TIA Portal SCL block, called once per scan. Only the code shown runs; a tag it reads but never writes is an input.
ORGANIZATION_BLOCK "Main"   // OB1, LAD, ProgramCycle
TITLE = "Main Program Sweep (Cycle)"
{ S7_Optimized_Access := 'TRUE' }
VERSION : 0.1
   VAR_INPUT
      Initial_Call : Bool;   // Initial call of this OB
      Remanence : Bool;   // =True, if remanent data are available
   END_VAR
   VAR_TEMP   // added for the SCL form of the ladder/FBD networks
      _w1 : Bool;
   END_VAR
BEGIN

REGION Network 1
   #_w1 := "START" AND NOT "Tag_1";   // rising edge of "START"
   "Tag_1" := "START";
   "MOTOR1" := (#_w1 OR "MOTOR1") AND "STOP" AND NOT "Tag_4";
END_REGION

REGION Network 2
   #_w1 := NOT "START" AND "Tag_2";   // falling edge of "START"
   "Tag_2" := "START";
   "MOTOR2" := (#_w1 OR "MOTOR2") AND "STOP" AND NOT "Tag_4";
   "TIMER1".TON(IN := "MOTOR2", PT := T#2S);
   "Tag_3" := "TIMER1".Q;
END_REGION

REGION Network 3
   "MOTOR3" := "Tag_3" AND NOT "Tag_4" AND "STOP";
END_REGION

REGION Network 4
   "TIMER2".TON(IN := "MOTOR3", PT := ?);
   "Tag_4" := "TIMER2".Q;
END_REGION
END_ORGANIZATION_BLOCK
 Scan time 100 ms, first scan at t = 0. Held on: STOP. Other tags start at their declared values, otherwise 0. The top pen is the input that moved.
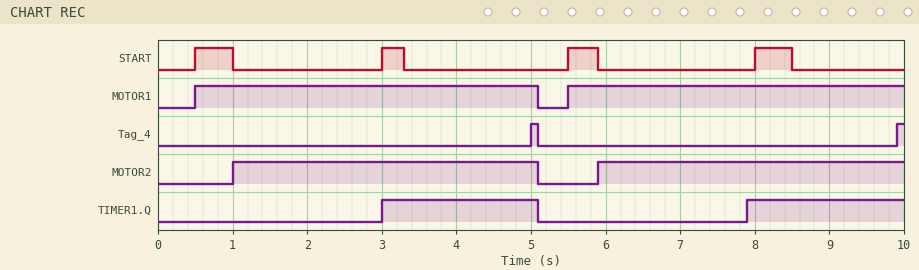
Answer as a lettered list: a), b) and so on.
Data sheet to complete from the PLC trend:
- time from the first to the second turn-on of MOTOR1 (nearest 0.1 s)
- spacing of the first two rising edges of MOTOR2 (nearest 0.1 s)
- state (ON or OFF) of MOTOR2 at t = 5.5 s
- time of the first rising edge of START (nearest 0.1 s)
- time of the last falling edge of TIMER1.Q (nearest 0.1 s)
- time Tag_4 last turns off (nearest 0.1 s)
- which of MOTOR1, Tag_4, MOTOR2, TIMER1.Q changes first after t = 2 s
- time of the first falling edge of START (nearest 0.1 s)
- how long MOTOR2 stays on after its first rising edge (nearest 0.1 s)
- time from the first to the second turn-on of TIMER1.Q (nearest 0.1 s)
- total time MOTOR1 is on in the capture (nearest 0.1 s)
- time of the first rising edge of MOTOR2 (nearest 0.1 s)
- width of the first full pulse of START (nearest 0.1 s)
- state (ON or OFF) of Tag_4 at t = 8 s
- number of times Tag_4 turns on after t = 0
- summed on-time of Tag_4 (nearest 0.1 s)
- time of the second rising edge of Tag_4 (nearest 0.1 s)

a) 5.0 s
b) 4.9 s
c) OFF
d) 0.5 s
e) 5.1 s
f) 5.1 s
g) TIMER1.Q
h) 1.0 s
i) 4.1 s
j) 4.9 s
k) 9.1 s
l) 1.0 s
m) 0.5 s
n) OFF
o) 2
p) 0.2 s
q) 9.9 s
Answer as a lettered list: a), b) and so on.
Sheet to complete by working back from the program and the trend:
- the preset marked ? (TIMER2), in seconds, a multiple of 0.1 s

a) 2.0 s
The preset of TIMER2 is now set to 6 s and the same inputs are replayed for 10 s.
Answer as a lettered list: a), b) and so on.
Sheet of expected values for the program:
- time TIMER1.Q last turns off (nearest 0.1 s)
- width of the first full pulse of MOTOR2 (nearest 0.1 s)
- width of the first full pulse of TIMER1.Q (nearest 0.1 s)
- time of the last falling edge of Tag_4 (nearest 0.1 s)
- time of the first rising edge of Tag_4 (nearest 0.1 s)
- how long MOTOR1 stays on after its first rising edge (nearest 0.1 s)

a) 9.1 s
b) 8.1 s
c) 6.1 s
d) 9.1 s
e) 9.0 s
f) 8.6 s
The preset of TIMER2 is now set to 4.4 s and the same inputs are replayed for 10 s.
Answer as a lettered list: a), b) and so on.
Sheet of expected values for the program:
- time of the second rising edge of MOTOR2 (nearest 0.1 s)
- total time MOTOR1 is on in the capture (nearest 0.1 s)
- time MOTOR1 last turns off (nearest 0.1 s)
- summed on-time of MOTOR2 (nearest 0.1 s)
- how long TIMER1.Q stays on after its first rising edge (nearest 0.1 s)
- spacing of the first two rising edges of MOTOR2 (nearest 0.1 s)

a) 8.5 s
b) 9.0 s
c) 7.5 s
d) 8.0 s
e) 4.5 s
f) 7.5 s
